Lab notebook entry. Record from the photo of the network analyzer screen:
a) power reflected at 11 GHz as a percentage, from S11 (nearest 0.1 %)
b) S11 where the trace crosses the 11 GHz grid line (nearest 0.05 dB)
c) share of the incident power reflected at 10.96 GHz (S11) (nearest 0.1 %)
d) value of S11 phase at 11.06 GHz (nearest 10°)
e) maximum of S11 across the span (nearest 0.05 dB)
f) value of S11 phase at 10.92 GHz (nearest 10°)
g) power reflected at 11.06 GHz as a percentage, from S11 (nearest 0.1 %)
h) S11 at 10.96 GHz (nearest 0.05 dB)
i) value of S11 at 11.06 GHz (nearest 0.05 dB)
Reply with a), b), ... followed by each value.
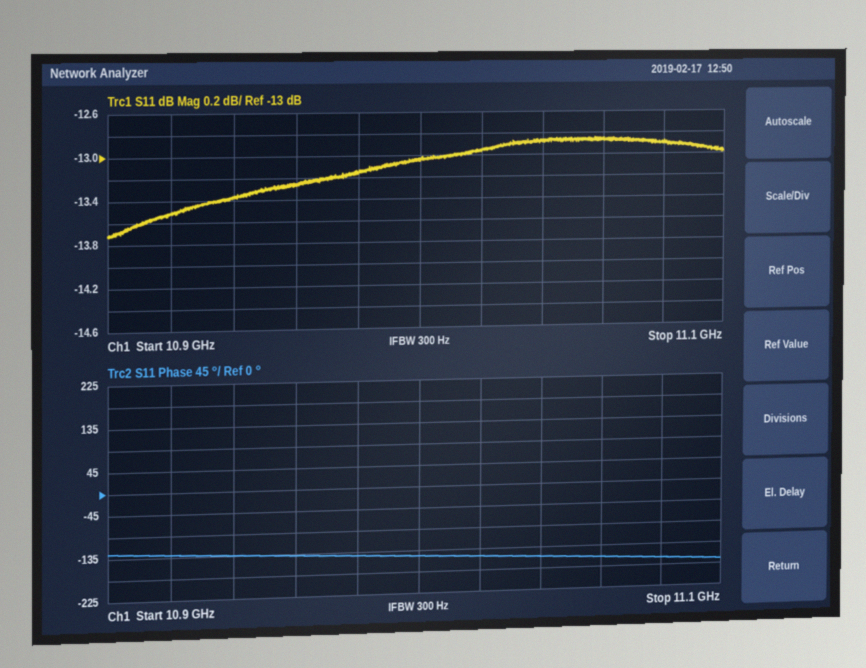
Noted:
a) 5.0 %
b) -13.05 dB
c) 4.7 %
d) -160°
e) -12.85 dB
f) -130°
g) 5.2 %
h) -13.25 dB
i) -12.85 dB
